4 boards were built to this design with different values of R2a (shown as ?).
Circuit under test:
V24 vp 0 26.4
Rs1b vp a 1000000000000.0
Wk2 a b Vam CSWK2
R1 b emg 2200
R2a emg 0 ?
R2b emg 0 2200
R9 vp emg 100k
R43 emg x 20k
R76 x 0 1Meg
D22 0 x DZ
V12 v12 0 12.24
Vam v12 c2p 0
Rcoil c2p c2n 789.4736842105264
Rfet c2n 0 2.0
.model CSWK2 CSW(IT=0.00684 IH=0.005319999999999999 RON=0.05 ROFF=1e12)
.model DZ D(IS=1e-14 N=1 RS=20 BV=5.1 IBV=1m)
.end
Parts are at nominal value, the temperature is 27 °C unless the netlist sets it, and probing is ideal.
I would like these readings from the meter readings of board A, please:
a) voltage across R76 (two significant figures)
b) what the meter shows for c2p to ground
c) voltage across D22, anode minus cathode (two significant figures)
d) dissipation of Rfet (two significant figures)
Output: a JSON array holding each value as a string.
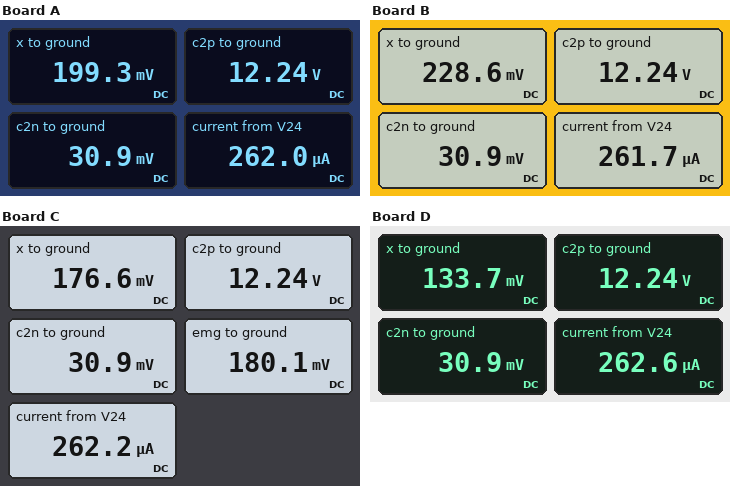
["200 mV", "12.24 V", "-200 mV", "480 µW"]
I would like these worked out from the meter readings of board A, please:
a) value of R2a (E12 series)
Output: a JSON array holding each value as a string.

["1.2 kΩ"]
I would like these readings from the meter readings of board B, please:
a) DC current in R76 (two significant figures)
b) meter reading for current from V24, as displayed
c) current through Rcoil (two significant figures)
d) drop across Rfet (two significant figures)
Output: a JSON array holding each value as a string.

["230 nA", "261.7 µA", "15 mA", "31 mV"]
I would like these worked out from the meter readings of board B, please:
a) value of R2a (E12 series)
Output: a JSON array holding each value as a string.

["1.5 kΩ"]
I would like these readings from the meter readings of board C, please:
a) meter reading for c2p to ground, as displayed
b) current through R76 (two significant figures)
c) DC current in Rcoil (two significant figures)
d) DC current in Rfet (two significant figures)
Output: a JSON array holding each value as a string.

["12.24 V", "180 nA", "15 mA", "15 mA"]
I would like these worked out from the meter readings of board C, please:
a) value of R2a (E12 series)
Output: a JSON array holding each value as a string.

["1 kΩ"]
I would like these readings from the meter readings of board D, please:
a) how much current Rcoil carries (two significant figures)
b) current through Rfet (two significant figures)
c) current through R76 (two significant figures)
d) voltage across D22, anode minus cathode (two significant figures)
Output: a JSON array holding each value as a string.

["15 mA", "15 mA", "130 nA", "-130 mV"]
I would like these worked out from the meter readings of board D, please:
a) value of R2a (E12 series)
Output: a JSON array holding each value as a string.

["680 Ω"]
